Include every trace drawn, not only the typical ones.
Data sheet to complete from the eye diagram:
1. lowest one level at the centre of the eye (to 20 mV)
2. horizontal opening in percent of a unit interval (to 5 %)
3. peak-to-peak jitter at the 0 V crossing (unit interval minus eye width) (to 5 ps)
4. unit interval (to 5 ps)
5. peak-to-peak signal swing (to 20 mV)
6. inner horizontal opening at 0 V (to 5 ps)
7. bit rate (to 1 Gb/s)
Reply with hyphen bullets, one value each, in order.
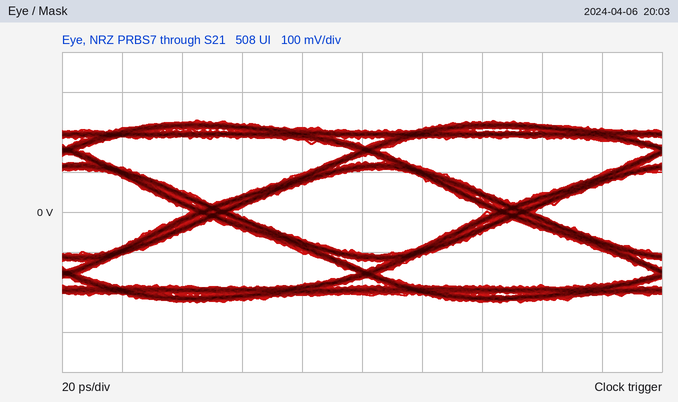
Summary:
- 100 mV
- 85 %
- 15 ps
- 100 ps
- 460 mV
- 85 ps
- 10 Gb/s
